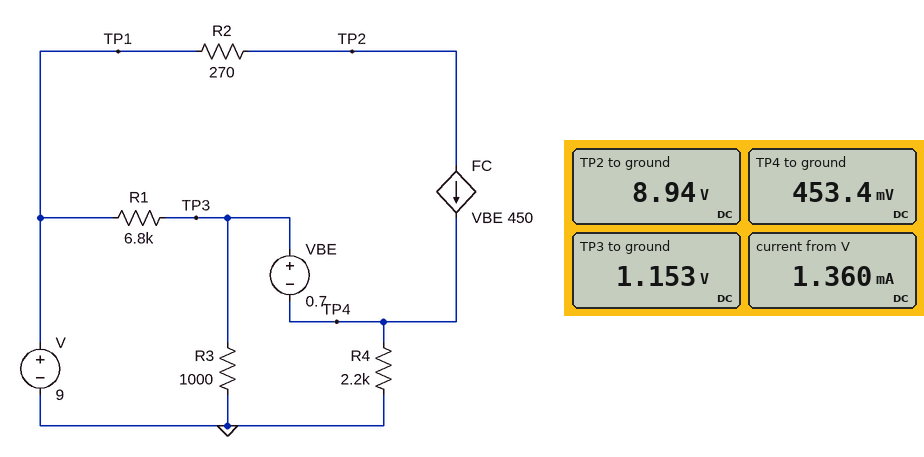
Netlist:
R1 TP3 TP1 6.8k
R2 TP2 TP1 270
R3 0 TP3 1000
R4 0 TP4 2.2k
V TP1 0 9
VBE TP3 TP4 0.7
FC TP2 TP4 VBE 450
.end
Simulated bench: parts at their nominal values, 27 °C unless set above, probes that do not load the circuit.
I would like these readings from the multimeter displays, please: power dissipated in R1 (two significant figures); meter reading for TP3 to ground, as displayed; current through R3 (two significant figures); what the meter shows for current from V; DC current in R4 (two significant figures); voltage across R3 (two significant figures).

9.1 mW
1.153 V
1.2 mA
1.360 mA
210 µA
1.2 V
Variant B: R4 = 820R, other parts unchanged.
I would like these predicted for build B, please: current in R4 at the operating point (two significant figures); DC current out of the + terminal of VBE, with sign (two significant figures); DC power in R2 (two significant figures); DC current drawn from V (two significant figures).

550 µA
-1.2 µA
82 µW
1.7 mA
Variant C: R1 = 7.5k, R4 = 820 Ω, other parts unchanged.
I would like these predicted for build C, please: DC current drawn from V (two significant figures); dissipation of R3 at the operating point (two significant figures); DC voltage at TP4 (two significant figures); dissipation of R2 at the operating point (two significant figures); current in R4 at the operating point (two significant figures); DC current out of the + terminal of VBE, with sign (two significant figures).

1.5 mA
1.1 mW
360 mV
51 µW
440 µA
-970 nA
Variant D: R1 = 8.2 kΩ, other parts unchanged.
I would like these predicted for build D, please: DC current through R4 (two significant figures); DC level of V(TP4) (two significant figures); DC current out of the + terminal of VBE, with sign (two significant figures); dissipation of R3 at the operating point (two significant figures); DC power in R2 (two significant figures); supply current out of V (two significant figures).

130 µA
280 mV
-280 nA
960 µW
4.3 µW
1.1 mA
